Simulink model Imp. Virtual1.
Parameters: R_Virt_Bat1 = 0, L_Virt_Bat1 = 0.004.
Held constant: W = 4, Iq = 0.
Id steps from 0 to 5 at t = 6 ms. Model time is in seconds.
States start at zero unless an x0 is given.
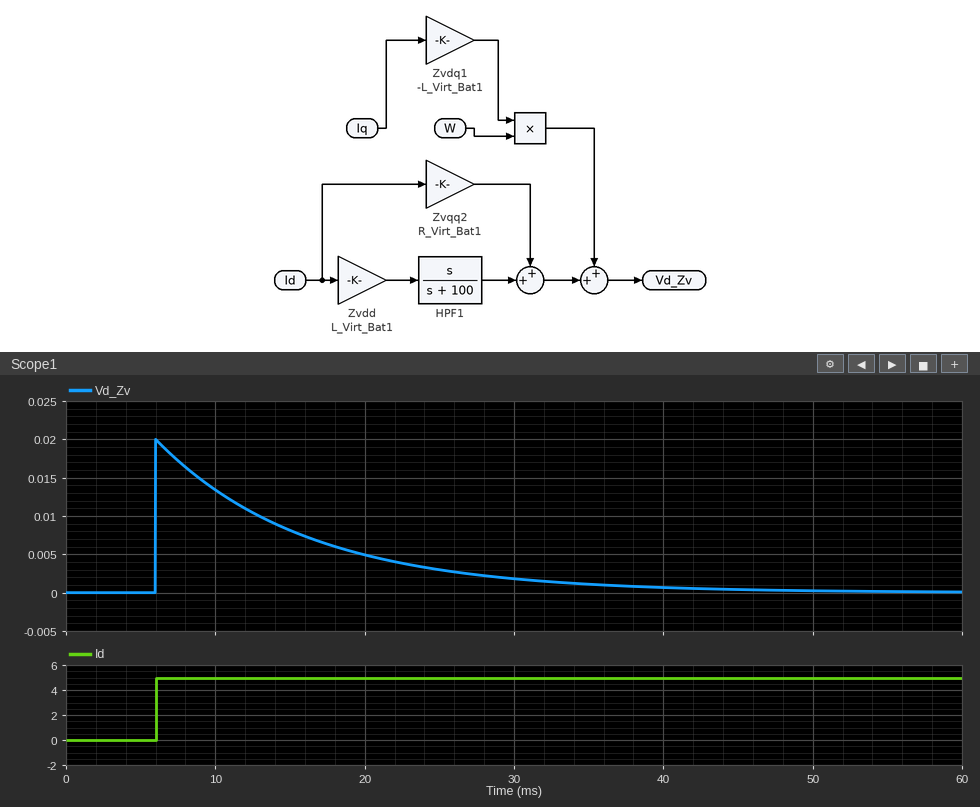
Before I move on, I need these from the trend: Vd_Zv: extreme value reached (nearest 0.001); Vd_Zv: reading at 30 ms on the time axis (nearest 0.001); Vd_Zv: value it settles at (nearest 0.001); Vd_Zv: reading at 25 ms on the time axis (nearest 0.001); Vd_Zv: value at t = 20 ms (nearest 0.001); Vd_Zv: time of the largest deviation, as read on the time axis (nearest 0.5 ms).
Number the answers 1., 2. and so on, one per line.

1. 0.020
2. 0.002
3. 0.000
4. 0.003
5. 0.005
6. 6.0 ms
